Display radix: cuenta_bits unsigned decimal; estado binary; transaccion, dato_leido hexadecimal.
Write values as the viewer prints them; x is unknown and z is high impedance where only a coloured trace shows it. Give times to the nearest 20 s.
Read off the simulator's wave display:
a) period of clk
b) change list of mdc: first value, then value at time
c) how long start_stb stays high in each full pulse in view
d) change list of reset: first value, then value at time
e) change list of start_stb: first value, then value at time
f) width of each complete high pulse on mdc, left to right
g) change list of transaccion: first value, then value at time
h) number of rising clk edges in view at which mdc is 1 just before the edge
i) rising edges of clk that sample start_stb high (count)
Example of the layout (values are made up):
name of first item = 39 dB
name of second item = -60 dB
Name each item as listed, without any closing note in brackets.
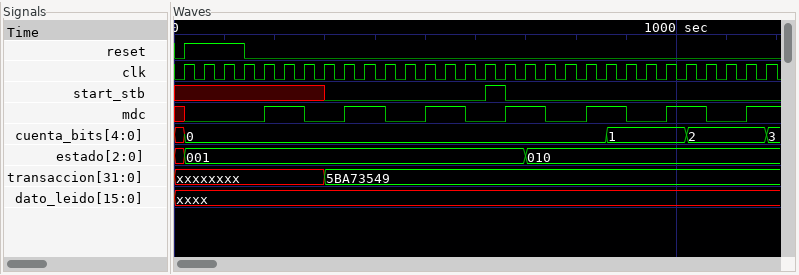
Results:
period of clk = 40 s
change list of mdc: first value, then value at time = x, 0 at 20 s, 1 at 180 s, 0 at 260 s, 1 at 340 s, 0 at 420 s, 1 at 500 s, 0 at 580 s, 1 at 660 s, 0 at 740 s, 1 at 820 s, 0 at 900 s, 1 at 980 s, 0 at 1060 s, 1 at 1140 s
how long start_stb stays high in each full pulse in view = 40 s
change list of reset: first value, then value at time = 0, 1 at 20 s, 0 at 140 s
change list of start_stb: first value, then value at time = x, 0 at 300 s, 1 at 620 s, 0 at 660 s
width of each complete high pulse on mdc, left to right = 80 s, 80 s, 80 s, 80 s, 80 s, 80 s
change list of transaccion: first value, then value at time = xxxxxxxx, 5BA73549 at 300 s
number of rising clk edges in view at which mdc is 1 just before the edge = 13
rising edges of clk that sample start_stb high = 1
